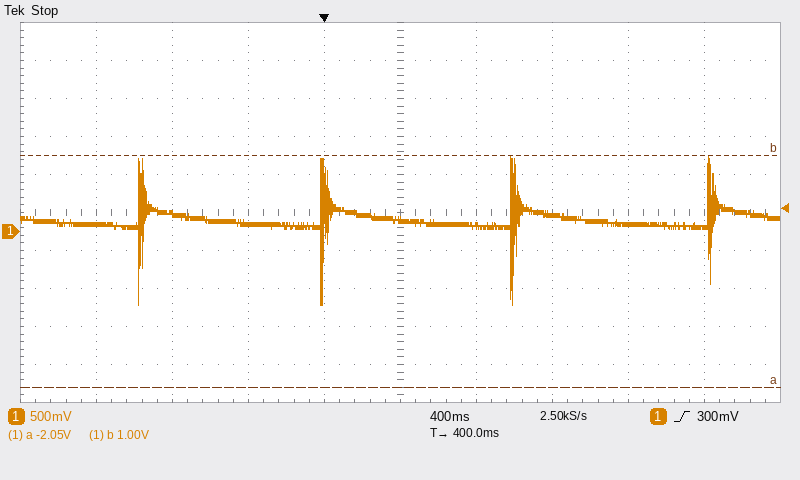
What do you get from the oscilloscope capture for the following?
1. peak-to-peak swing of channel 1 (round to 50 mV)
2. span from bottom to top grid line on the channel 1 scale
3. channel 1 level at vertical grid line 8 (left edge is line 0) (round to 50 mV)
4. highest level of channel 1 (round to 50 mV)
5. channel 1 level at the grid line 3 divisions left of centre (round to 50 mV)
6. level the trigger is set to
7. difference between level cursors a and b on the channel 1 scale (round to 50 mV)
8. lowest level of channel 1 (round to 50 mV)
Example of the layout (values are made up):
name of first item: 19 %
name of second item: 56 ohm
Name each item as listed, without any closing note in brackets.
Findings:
peak-to-peak swing of channel 1: 1.95 V
span from bottom to top grid line on the channel 1 scale: 5 V
channel 1 level at vertical grid line 8 (left edge is line 0): 100 mV
highest level of channel 1: 1.00 V
channel 1 level at the grid line 3 divisions left of centre: 250 mV
level the trigger is set to: 300 mV
difference between level cursors a and b on the channel 1 scale: 3.05 V
lowest level of channel 1: -950 mV
